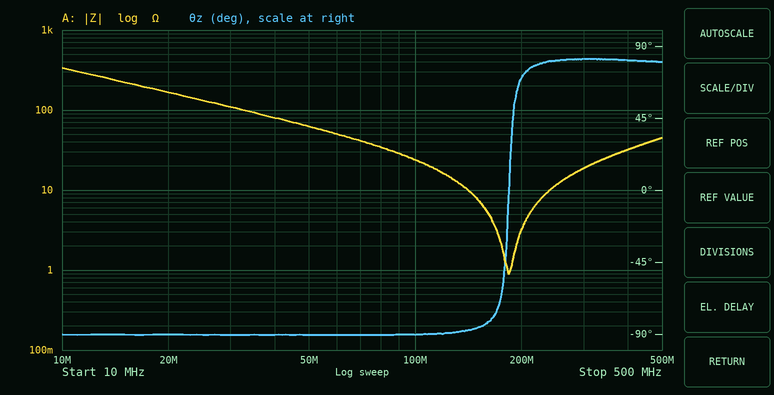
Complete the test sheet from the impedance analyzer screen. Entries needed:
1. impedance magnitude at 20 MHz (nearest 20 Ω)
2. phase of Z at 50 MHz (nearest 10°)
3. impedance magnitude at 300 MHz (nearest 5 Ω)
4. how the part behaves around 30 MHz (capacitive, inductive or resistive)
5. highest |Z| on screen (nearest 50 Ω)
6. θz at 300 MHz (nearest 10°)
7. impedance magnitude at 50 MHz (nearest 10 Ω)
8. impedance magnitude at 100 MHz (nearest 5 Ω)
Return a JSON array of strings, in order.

["160 Ω", "-90°", "20 Ω", "capacitive", "350 Ω", "80°", "60 Ω", "25 Ω"]
